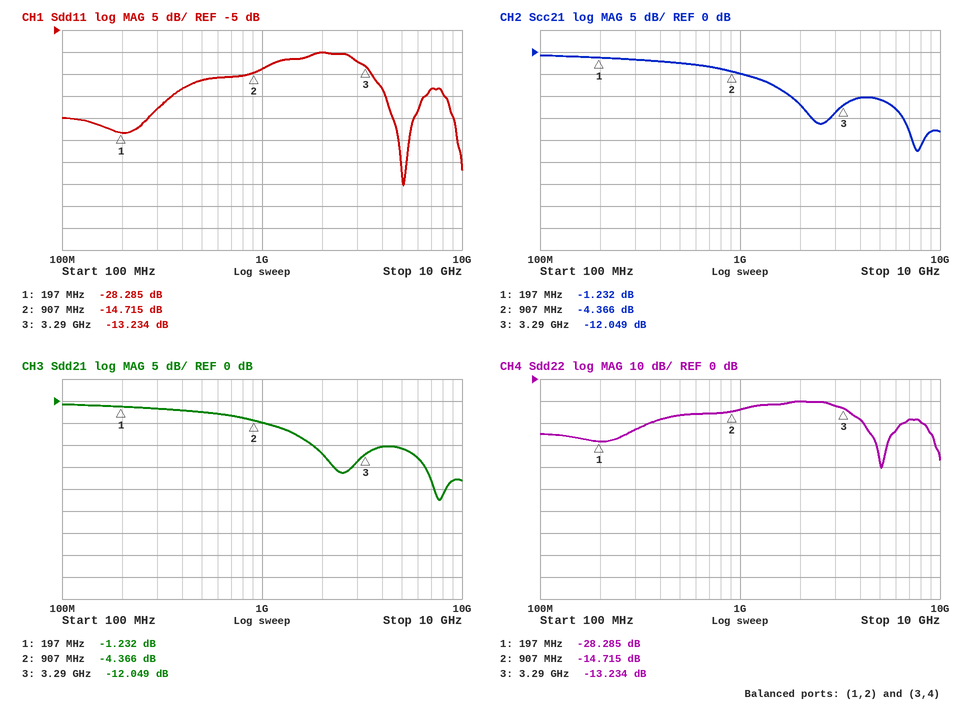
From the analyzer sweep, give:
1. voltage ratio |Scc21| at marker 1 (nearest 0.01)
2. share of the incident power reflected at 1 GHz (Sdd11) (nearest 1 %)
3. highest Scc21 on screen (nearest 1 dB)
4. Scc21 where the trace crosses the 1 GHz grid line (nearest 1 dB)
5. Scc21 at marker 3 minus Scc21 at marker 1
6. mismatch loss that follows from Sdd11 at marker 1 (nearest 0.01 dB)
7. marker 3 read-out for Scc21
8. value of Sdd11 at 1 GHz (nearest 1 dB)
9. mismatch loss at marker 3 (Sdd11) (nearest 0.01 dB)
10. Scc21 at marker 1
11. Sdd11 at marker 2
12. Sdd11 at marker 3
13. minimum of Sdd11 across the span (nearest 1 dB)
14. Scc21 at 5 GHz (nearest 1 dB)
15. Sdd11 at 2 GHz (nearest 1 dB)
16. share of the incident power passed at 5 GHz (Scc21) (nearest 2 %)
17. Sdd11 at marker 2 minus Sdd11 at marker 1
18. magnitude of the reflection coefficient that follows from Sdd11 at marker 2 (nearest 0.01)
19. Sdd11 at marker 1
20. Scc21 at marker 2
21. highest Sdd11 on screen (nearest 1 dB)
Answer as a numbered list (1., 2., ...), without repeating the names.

1. 0.87
2. 4 %
3. -1 dB
4. -5 dB
5. -10.817 dB
6. 0.01 dB
7. -12.049 dB
8. -14 dB
9. 0.21 dB
10. -1.232 dB
11. -14.715 dB
12. -13.234 dB
13. -40 dB
14. -11 dB
15. -10 dB
16. 8 %
17. 13.570 dB
18. 0.18
19. -28.285 dB
20. -4.366 dB
21. -10 dB
